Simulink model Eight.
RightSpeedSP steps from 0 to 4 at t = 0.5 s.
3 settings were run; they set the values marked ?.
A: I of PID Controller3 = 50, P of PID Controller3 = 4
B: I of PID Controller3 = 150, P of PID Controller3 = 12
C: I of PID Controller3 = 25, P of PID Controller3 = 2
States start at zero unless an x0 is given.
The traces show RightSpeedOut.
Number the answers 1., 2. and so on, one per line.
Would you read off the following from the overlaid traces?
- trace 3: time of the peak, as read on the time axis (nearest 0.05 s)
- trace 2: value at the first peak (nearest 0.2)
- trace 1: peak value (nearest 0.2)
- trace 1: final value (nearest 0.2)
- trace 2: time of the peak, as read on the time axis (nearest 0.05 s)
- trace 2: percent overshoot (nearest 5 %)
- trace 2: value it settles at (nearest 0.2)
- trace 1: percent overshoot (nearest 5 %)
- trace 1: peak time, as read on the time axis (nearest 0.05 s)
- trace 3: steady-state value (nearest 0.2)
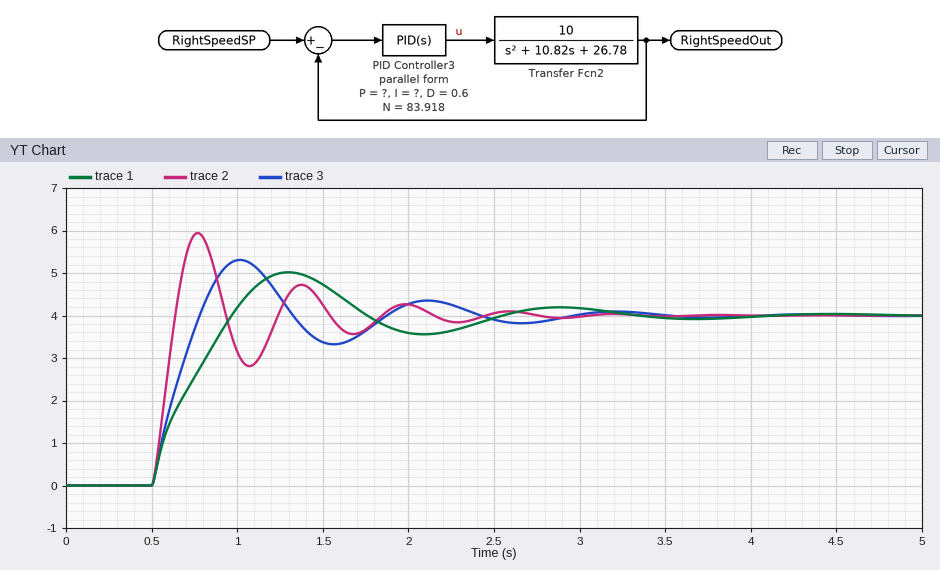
1. 1.00 s
2. 6.0
3. 5.0
4. 4.0
5. 0.75 s
6. 50 %
7. 4.0
8. 25 %
9. 1.30 s
10. 4.0
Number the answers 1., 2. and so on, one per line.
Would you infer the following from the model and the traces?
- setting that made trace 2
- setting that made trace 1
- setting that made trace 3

1. B
2. C
3. A
